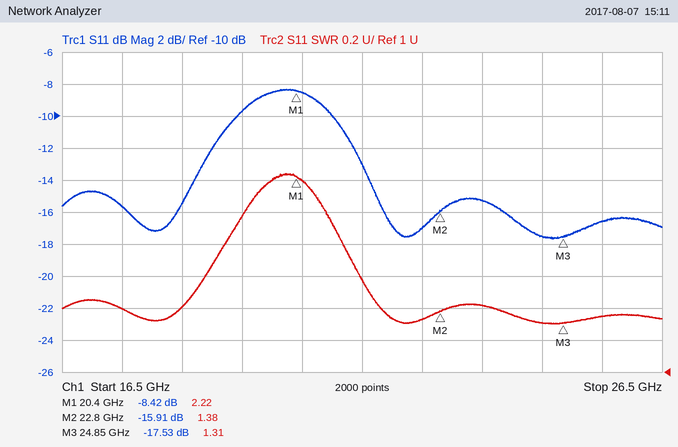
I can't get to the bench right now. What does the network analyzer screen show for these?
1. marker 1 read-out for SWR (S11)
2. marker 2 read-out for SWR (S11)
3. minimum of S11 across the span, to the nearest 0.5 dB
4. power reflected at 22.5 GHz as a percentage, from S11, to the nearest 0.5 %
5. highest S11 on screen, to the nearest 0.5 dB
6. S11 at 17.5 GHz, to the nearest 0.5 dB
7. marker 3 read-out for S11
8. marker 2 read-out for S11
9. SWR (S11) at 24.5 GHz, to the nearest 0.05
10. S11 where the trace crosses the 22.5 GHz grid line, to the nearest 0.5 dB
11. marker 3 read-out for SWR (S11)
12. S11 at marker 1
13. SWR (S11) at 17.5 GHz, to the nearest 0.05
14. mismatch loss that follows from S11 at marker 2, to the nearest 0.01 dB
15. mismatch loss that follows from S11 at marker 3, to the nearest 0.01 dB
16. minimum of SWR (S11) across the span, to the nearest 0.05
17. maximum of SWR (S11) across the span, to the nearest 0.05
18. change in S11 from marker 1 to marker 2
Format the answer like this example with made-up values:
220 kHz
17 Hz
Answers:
2.22
1.38
-17.5 dB
2.0 %
-8.5 dB
-15.5 dB
-17.53 dB
-15.91 dB
1.30
-17.0 dB
1.31
-8.42 dB
1.40
0.11 dB
0.08 dB
1.30
2.25
-7.49 dB
